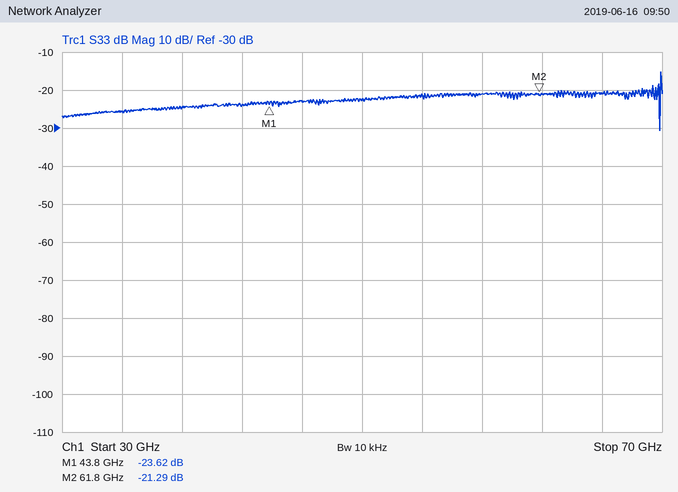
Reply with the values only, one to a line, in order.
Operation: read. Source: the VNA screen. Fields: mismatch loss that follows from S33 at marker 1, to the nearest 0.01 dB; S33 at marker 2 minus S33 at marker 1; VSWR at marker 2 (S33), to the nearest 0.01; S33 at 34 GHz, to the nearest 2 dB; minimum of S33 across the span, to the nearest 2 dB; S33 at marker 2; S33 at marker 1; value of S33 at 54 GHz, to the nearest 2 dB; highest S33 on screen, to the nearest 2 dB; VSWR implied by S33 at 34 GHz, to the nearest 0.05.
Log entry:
0.02 dB
2.33 dB
1.19
-26 dB
-30 dB
-21.29 dB
-23.62 dB
-22 dB
-16 dB
1.10
